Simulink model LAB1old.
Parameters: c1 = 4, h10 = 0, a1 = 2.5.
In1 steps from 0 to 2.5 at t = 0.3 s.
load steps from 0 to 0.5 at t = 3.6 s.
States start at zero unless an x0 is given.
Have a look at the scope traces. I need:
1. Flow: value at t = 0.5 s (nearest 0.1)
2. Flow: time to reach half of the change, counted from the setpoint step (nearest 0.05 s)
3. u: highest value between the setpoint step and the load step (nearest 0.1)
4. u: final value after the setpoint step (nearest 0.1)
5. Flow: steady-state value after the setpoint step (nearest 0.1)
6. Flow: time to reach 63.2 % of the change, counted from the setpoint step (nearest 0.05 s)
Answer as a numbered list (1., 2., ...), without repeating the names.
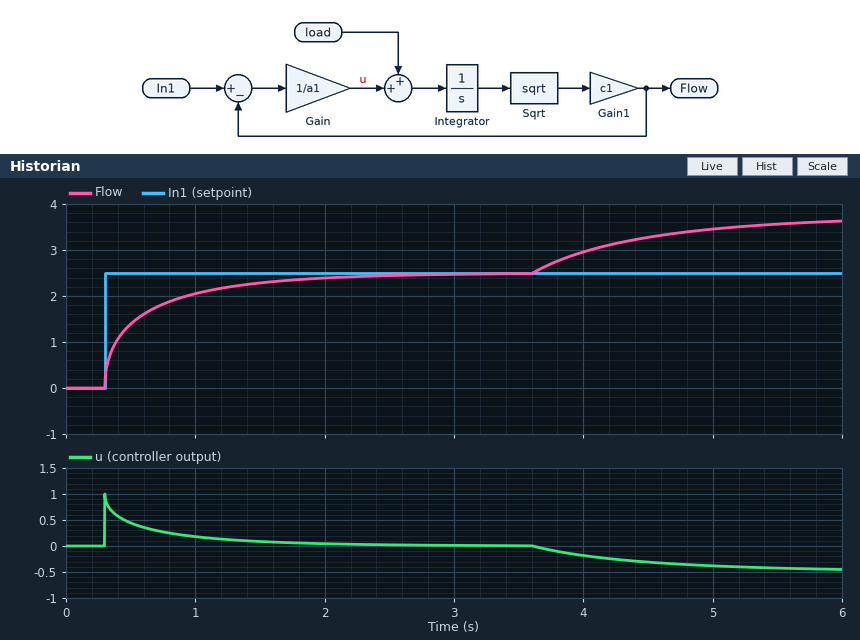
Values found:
1. 1.4
2. 0.15 s
3. 1.0
4. 0.0
5. 2.5
6. 0.30 s
